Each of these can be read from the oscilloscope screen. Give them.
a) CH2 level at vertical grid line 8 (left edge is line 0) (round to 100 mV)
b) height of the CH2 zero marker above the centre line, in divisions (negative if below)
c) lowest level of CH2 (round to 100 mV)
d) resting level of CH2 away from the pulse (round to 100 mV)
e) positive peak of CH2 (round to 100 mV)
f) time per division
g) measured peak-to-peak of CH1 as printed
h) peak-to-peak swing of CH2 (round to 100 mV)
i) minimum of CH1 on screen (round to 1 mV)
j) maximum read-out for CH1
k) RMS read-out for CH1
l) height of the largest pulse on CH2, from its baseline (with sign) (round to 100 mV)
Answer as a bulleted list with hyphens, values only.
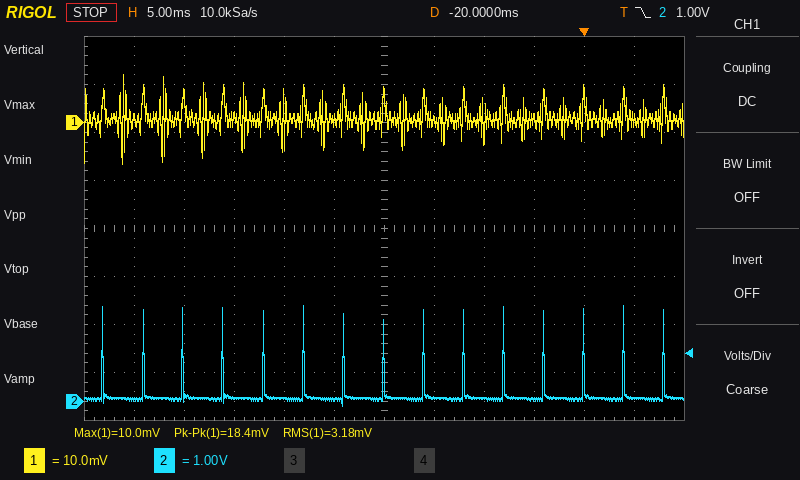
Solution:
- 100 mV
- -3.6 div
- -100 mV
- 100 mV
- 2.0 V
- 5 ms
- 18.4 mV
- 2.1 V
- -8 mV
- 10.0 mV
- 3.18 mV
- +1.9 V
